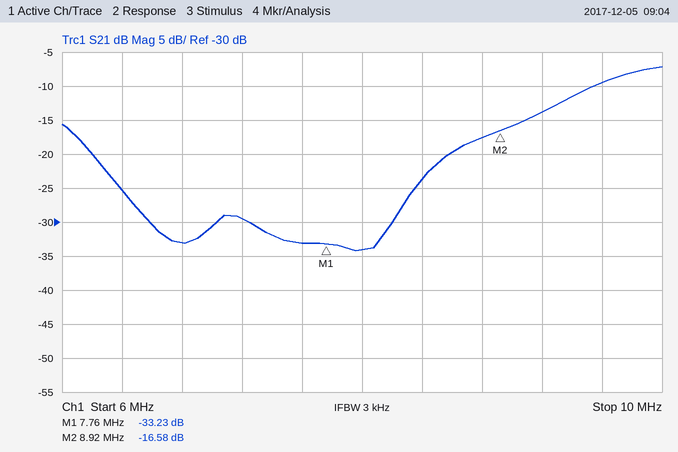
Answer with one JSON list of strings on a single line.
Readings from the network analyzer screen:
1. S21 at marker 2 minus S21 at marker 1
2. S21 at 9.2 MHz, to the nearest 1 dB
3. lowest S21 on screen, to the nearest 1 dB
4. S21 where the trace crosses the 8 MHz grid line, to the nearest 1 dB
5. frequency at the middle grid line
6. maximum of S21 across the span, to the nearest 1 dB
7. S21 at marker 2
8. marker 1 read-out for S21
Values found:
["16.65 dB", "-14 dB", "-34 dB", "-34 dB", "8 MHz", "-7 dB", "-16.58 dB", "-33.23 dB"]
